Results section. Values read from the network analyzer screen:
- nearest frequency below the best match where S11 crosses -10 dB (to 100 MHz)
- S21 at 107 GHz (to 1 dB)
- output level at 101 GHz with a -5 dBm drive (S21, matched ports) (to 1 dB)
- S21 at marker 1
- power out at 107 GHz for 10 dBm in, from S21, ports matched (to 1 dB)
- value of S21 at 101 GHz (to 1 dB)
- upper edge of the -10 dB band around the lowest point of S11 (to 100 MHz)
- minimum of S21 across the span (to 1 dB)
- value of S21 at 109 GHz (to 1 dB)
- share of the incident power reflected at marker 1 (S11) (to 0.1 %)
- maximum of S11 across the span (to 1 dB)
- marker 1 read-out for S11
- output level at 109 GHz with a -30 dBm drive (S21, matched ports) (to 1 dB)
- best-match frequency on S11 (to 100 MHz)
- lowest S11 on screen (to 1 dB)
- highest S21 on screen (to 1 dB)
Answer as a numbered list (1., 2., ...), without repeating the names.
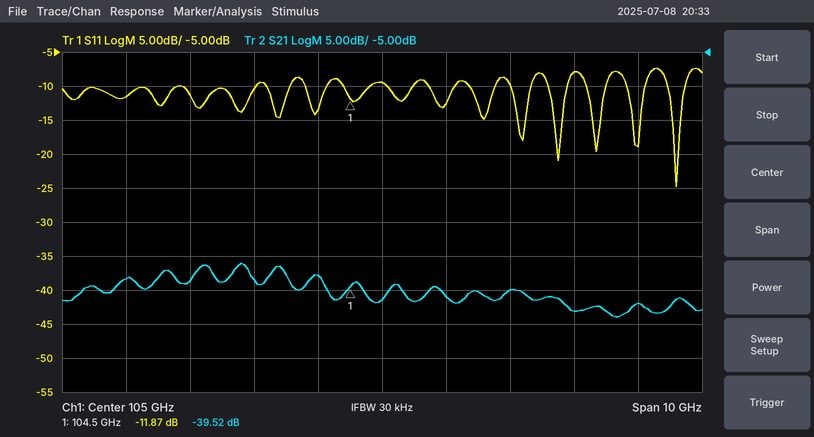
1. 109.5 GHz
2. -40 dB
3. -43 dBm
4. -39.52 dB
5. -30 dBm
6. -38 dB
7. 109.7 GHz
8. -44 dB
9. -42 dB
10. 6.5 %
11. -7 dB
12. -11.87 dB
13. -72 dBm
14. 109.6 GHz
15. -25 dB
16. -36 dB
